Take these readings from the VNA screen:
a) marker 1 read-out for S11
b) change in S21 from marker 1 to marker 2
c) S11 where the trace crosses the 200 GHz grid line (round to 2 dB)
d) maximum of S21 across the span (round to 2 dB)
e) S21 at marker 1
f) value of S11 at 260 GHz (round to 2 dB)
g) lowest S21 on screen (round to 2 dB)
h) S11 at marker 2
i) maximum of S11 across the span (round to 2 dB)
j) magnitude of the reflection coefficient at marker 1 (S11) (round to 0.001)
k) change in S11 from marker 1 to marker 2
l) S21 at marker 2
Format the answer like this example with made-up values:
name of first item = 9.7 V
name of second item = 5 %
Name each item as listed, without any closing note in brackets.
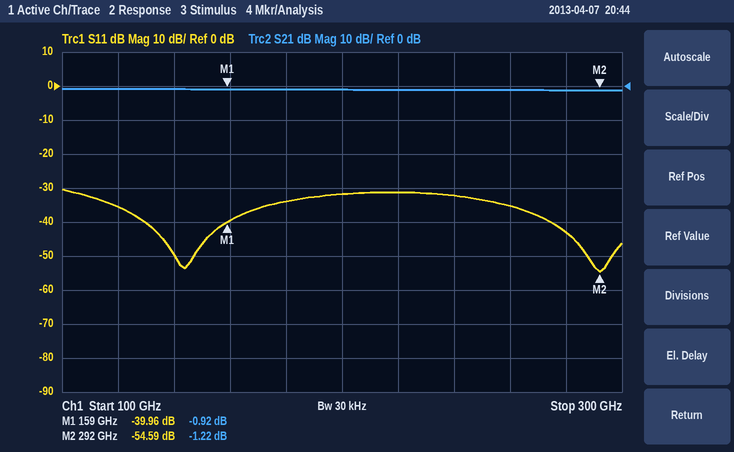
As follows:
marker 1 read-out for S11 = -39.96 dB
change in S21 from marker 1 to marker 2 = -0.30 dB
S11 where the trace crosses the 200 GHz grid line = -32 dB
maximum of S21 across the span = 0 dB
S21 at marker 1 = -0.92 dB
value of S11 at 260 GHz = -36 dB
lowest S21 on screen = -2 dB
S11 at marker 2 = -54.59 dB
maximum of S11 across the span = -30 dB
magnitude of the reflection coefficient at marker 1 (S11) = 0.010
change in S11 from marker 1 to marker 2 = -14.63 dB
S21 at marker 2 = -1.22 dB
